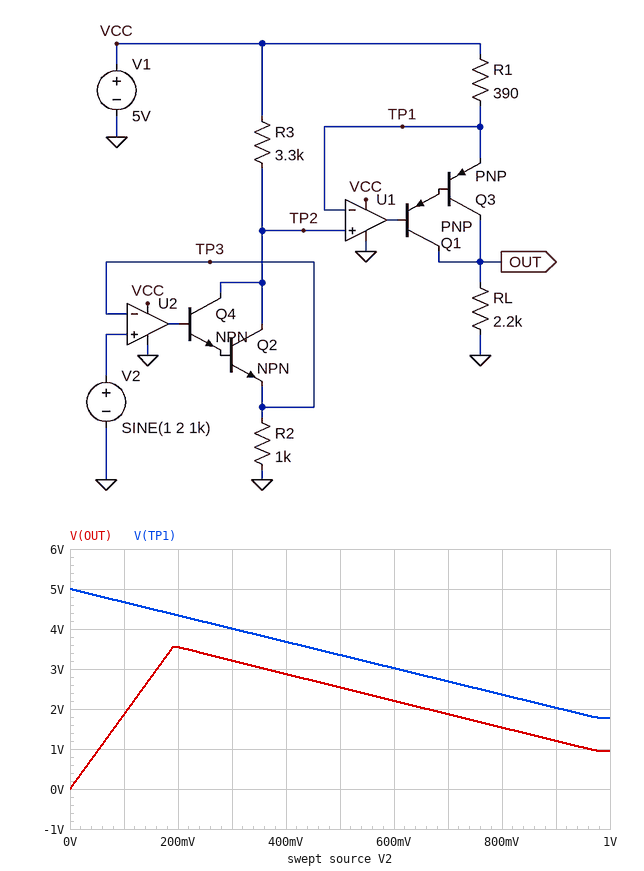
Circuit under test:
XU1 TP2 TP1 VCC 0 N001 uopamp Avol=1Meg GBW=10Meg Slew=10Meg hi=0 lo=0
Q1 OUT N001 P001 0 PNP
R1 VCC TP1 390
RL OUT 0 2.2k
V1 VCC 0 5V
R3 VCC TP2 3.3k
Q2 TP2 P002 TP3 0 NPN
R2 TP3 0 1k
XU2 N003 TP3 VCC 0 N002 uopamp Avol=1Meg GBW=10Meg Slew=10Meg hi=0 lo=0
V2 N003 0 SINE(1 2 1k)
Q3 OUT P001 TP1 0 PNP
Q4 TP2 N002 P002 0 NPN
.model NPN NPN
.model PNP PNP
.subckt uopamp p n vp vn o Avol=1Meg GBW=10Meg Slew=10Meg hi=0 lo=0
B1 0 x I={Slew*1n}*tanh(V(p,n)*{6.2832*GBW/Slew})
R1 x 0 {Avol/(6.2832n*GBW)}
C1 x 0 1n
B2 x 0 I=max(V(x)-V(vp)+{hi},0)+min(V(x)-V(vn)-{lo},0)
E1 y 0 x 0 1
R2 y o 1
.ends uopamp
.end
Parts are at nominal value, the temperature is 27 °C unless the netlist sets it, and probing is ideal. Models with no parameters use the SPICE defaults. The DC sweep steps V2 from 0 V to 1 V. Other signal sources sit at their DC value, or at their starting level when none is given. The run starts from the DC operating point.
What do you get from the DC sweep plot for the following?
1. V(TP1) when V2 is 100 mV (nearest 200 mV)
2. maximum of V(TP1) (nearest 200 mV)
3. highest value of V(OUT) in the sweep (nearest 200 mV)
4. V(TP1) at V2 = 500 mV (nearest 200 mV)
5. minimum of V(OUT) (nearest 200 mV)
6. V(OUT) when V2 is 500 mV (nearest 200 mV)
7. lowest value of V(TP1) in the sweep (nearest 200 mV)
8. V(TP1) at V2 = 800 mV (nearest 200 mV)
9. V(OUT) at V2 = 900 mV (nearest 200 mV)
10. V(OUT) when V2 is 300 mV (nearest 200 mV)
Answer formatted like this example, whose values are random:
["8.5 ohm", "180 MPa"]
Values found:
["4.6 V", "5.0 V", "3.6 V", "3.4 V", "0 V", "2.6 V", "1.8 V", "2.4 V", "1.2 V", "3.2 V"]
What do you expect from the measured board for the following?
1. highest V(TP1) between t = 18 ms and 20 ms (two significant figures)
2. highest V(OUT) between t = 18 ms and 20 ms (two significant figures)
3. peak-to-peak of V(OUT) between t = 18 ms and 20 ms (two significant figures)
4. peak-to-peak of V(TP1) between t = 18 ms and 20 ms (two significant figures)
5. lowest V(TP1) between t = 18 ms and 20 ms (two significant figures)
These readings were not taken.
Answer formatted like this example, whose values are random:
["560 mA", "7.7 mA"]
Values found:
["5.0 V", "3.6 V", "3.6 V", "3.2 V", "1.8 V"]
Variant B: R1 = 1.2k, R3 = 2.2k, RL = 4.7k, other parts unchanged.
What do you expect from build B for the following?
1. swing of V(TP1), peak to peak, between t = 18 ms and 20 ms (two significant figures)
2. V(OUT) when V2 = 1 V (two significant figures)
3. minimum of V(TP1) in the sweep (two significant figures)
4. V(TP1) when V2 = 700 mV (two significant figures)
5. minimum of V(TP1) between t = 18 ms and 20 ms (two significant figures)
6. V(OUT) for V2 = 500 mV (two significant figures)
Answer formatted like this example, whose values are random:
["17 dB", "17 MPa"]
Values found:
["2.9 V", "2.0 V", "2.8 V", "3.5 V", "2.1 V", "3.1 V"]
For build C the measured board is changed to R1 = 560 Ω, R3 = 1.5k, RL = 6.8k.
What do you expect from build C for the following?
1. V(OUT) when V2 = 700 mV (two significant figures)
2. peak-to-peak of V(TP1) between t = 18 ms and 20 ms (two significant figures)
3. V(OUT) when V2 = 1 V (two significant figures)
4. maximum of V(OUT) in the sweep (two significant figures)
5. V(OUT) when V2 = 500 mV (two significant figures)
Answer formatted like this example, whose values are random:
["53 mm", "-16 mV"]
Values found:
["3.2 V", "2.5 V", "2.7 V", "3.9 V", "3.5 V"]
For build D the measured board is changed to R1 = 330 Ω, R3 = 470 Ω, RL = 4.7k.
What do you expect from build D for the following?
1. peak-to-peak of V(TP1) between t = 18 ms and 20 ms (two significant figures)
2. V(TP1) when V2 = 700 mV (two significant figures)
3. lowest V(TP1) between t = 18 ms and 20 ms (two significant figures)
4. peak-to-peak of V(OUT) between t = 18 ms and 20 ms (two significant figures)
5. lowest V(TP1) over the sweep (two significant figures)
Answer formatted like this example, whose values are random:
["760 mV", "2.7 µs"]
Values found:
["1.3 V", "4.7 V", "3.7 V", "3.9 V", "4.5 V"]
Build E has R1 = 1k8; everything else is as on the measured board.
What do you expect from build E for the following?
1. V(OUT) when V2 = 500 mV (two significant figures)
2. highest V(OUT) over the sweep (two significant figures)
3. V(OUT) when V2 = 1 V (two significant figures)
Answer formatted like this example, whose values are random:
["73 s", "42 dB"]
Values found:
["2.0 V", "2.3 V", "990 mV"]
